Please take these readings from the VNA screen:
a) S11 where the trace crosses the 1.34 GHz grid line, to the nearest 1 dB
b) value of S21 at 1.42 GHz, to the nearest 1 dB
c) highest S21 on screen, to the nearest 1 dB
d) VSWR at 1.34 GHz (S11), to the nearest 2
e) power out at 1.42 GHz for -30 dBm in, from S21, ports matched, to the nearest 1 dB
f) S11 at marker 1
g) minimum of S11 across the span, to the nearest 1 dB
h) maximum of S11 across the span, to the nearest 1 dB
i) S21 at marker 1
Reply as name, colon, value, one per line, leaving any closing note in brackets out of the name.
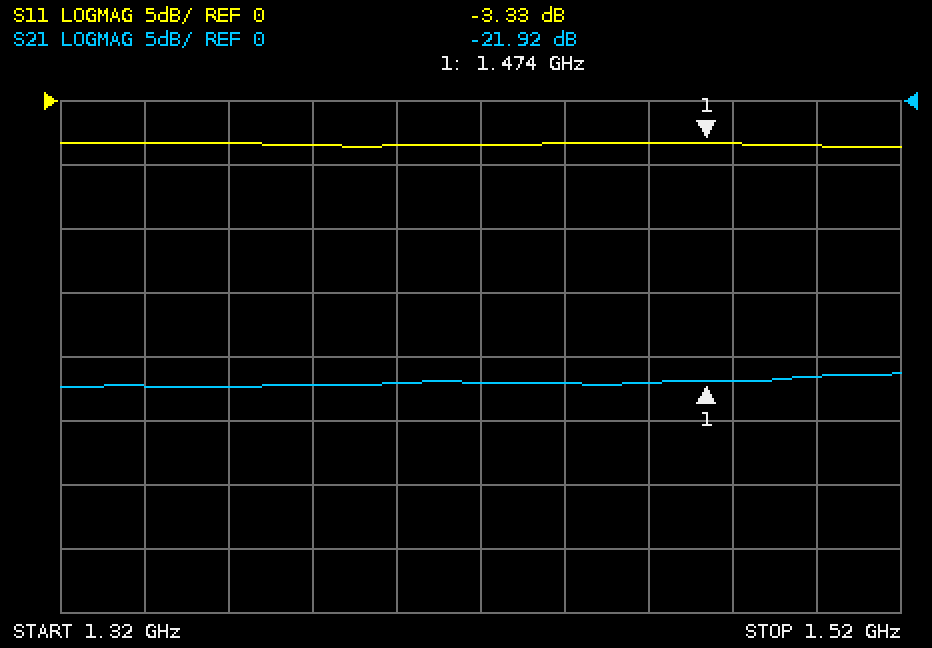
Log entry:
S11 where the trace crosses the 1.34 GHz grid line, to the nearest 1 dB: -3 dB
value of S21 at 1.42 GHz, to the nearest 1 dB: -22 dB
highest S21 on screen, to the nearest 1 dB: -21 dB
VSWR at 1.34 GHz (S11), to the nearest 2: 6
power out at 1.42 GHz for -30 dBm in, from S21, ports matched, to the nearest 1 dB: -52 dBm
S11 at marker 1: -3.33 dB
minimum of S11 across the span, to the nearest 1 dB: -4 dB
maximum of S11 across the span, to the nearest 1 dB: -3 dB
S21 at marker 1: -21.92 dB
